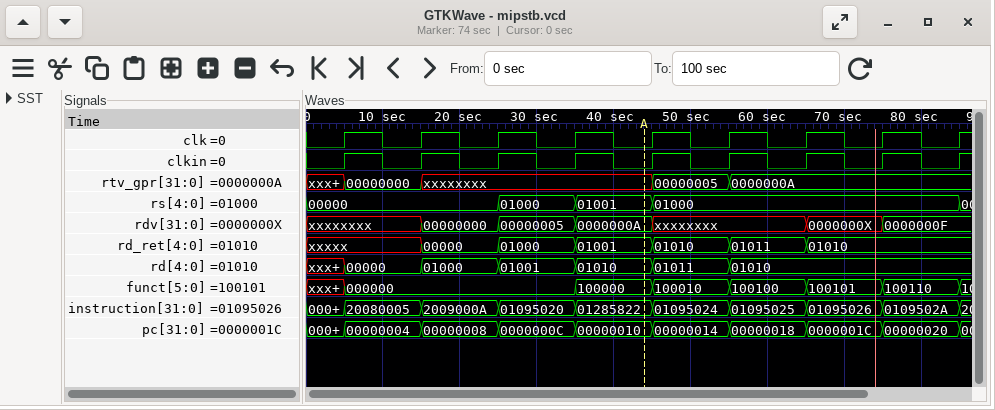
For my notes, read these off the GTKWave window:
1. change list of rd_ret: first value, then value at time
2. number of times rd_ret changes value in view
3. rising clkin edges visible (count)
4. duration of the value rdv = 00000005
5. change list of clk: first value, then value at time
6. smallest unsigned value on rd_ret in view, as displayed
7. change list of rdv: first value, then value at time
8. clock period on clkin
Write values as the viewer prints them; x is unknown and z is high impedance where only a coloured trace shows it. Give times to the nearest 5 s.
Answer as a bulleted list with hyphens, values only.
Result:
- xxxxx, 00000 at 15 s, 01000 at 25 s, 01001 at 35 s, 01010 at 45 s, 01011 at 55 s, 01010 at 65 s
- 6
- 9
- 10 s
- 0, 1 at 5 s, 0 at 10 s, 1 at 15 s, 0 at 20 s, 1 at 25 s, 0 at 30 s, 1 at 35 s, 0 at 40 s, 1 at 45 s, 0 at 50 s, 1 at 55 s, 0 at 60 s, 1 at 65 s, 0 at 70 s, 1 at 75 s, 0 at 80 s, 1 at 85 s
- 00000
- xxxxxxxx, 00000000 at 15 s, 00000005 at 25 s, 0000000A at 35 s, xxxxxxxx at 45 s, 0000000X at 65 s, 0000000F at 75 s
- 10 s
